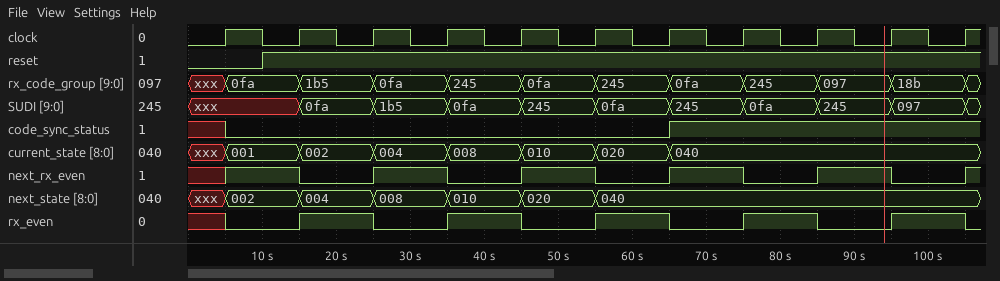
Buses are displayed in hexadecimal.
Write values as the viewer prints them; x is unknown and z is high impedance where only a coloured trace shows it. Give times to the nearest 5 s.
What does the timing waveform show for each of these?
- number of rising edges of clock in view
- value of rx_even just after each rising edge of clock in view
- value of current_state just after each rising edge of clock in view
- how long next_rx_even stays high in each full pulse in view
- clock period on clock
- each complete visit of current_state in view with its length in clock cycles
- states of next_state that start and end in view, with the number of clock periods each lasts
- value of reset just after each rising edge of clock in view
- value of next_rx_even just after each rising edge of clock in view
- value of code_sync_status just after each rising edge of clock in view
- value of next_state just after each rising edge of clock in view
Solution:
11
0 1 0 1 0 1 0 1 0 1 0
001, 002, 004, 008, 010, 020, 040, 040, 040, 040, 040
10 s, 10 s, 10 s, 10 s
10 s
001: 1, 002: 1, 004: 1, 008: 1, 010: 1, 020: 1
002: 1, 004: 1, 008: 1, 010: 1, 020: 1
0 1 1 1 1 1 1 1 1 1 1
1 0 1 0 1 0 1 0 1 0 1
0 0 0 0 0 0 1 1 1 1 1
002, 004, 008, 010, 020, 040, 040, 040, 040, 040, 040
